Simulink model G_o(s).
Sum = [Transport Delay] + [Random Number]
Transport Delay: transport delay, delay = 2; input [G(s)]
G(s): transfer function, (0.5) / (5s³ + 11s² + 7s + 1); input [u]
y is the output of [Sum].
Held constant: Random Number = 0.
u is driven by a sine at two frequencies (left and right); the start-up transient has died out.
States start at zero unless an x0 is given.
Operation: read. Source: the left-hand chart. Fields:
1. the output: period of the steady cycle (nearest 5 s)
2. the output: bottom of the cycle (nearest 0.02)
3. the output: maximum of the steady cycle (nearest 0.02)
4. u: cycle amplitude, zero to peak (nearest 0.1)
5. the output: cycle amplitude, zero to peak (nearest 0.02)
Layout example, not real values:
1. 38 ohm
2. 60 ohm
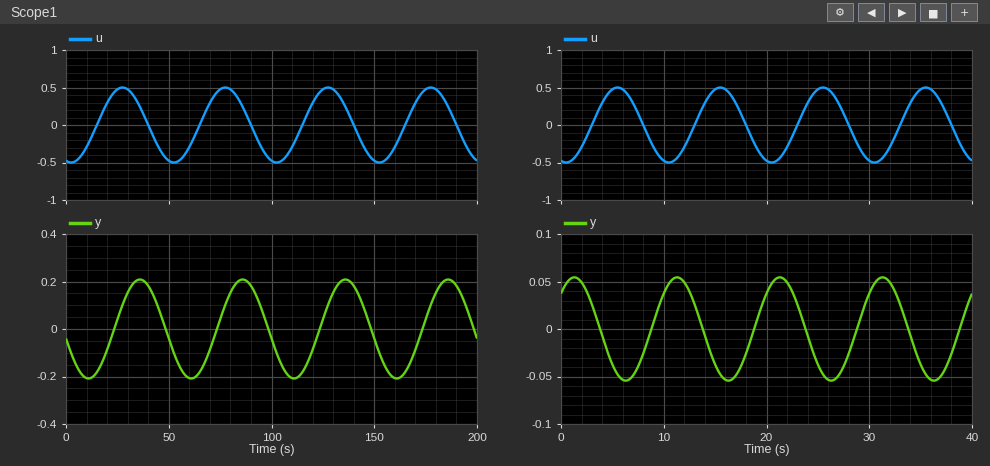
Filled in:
1. 50 s
2. -0.20
3. 0.20
4. 0.5
5. 0.20
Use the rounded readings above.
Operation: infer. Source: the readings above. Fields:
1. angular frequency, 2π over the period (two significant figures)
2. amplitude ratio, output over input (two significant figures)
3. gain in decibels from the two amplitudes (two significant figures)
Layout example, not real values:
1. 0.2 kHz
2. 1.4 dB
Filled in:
1. 0.13 rad/s
2. 0.40
3. -8.0 dB
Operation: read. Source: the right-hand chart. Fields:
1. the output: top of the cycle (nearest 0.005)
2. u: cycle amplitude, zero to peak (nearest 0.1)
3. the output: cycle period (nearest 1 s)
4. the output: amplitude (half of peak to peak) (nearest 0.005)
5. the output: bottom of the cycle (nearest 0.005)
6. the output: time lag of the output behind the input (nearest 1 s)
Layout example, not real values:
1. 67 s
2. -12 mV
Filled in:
1. 0.055
2. 0.5
3. 10 s
4. 0.055
5. -0.055
6. 6 s
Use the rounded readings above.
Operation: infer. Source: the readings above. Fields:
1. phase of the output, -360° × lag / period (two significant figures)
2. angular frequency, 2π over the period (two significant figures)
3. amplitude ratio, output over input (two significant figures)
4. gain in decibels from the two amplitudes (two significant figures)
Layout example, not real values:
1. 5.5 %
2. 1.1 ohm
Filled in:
1. -220°
2. 0.63 rad/s
3. 0.11
4. -19 dB
